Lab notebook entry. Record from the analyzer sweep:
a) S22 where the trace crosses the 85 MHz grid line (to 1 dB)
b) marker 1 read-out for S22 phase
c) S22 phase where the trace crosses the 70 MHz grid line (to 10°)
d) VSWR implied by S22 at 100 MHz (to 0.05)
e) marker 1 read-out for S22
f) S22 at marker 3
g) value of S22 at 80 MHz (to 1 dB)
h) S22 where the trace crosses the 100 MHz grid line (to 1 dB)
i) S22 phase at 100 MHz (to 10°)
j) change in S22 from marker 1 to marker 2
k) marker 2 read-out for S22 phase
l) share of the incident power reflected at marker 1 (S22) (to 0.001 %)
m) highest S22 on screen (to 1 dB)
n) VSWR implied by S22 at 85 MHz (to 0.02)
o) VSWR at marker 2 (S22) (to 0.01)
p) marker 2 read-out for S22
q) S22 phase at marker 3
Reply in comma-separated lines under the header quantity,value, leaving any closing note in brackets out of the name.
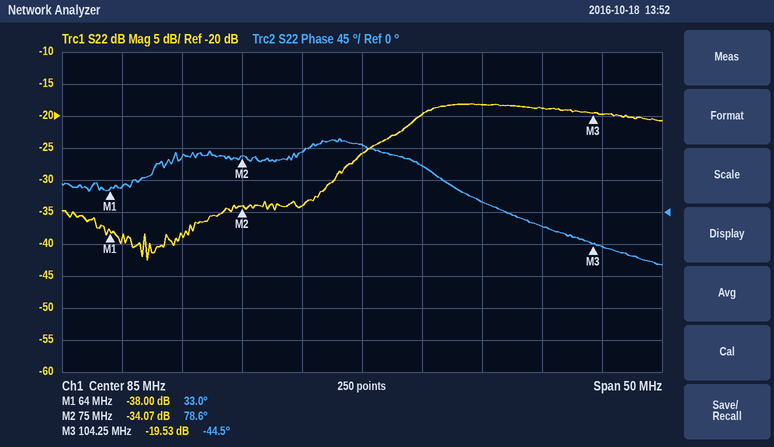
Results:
quantity,value
S22 where the trace crosses the 85 MHz grid line,-26 dB
marker 1 read-out for S22 phase,33.0°
S22 phase where the trace crosses the 70 MHz grid line,80°
VSWR implied by S22 at 100 MHz,1.25
marker 1 read-out for S22,-38.00 dB
S22 at marker 3,-19.53 dB
value of S22 at 80 MHz,-34 dB
S22 where the trace crosses the 100 MHz grid line,-19 dB
S22 phase at 100 MHz,-20°
change in S22 from marker 1 to marker 2,3.93 dB
marker 2 read-out for S22 phase,78.6°
share of the incident power reflected at marker 1 (S22),0.016 %
highest S22 on screen,-18 dB
VSWR implied by S22 at 85 MHz,1.10
VSWR at marker 2 (S22),1.04
marker 2 read-out for S22,-34.07 dB
S22 phase at marker 3,-44.5°
